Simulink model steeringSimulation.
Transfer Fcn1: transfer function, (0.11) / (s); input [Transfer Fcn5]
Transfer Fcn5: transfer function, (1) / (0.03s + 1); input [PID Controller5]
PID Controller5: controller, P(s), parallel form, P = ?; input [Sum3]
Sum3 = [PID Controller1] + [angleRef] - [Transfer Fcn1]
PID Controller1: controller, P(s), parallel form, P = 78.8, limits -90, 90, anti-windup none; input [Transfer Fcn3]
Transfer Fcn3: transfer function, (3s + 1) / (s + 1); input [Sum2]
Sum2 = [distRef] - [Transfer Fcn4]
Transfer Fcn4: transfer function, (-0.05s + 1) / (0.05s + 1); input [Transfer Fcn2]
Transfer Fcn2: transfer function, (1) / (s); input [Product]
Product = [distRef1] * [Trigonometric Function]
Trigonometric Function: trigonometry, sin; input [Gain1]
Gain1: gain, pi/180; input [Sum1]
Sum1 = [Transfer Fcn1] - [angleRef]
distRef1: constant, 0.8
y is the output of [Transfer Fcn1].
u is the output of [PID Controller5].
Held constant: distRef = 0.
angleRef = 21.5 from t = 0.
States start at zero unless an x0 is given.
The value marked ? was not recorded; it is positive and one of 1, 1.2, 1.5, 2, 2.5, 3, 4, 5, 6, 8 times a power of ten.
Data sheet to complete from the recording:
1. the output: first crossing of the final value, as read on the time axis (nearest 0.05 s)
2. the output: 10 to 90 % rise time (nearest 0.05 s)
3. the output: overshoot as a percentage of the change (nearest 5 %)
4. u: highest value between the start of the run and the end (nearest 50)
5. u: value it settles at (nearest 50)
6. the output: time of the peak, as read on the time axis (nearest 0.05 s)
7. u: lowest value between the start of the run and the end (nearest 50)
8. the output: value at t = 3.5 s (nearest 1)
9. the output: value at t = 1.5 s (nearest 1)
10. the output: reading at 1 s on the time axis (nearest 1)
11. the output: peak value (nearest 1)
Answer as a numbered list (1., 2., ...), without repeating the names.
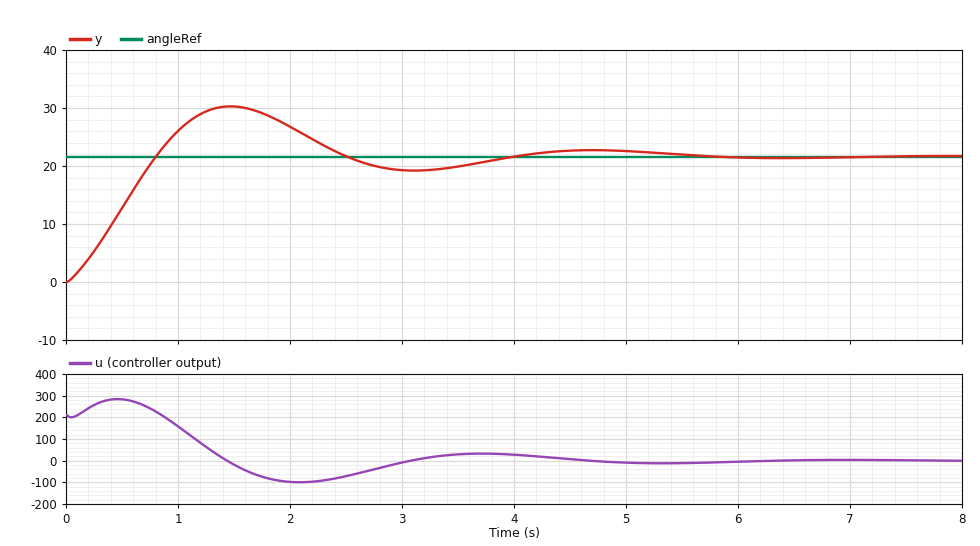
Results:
1. 0.80 s
2. 0.60 s
3. 40 %
4. 300
5. 0
6. 1.45 s
7. -100
8. 20
9. 30
10. 26
11. 30
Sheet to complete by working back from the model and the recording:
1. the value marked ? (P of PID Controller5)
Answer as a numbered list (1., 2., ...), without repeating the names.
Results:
1. 10
